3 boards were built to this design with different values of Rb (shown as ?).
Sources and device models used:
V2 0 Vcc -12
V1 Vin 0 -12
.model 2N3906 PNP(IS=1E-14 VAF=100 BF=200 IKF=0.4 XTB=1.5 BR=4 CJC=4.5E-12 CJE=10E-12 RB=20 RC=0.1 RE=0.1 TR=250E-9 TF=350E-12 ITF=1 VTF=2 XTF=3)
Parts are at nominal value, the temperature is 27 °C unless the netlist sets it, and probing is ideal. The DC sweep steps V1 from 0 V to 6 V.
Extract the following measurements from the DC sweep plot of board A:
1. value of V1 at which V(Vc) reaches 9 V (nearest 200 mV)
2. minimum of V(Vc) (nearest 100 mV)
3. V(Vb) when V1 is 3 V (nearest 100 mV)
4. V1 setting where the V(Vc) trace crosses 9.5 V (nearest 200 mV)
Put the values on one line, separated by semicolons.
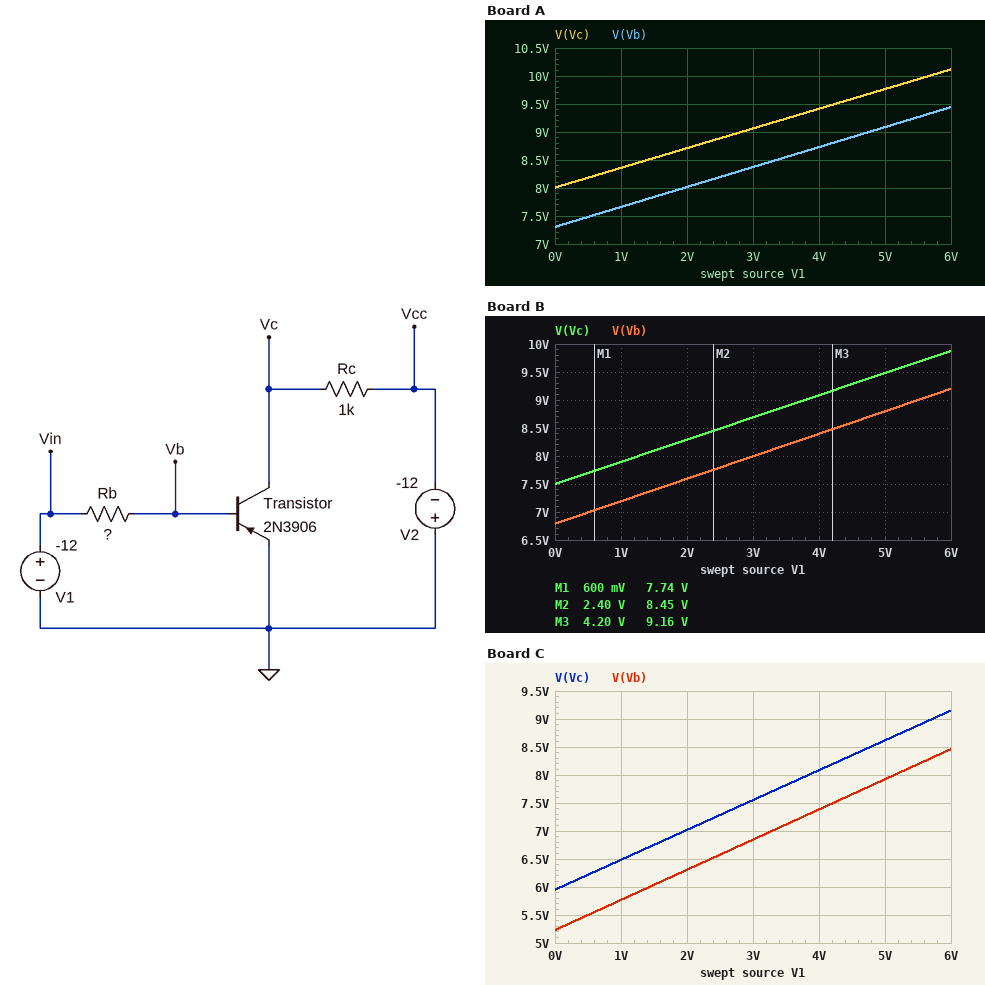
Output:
2.8 V; 8.0 V; 8.4 V; 4.2 V
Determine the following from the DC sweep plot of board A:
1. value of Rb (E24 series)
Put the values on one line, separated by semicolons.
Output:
9.1 kΩ
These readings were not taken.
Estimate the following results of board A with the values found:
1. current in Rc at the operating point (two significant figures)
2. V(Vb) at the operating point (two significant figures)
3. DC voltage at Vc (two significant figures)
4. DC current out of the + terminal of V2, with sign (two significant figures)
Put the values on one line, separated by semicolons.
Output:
8.2 mA; 3.0 V; 3.8 V; -8.2 mA
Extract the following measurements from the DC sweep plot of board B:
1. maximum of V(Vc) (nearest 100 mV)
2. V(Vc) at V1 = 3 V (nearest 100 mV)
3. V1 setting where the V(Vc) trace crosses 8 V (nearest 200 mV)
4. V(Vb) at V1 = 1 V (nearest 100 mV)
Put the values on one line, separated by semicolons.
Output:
9.9 V; 8.7 V; 1.2 V; 7.2 V
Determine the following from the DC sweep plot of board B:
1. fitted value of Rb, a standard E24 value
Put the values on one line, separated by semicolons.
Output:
7.5 kΩ
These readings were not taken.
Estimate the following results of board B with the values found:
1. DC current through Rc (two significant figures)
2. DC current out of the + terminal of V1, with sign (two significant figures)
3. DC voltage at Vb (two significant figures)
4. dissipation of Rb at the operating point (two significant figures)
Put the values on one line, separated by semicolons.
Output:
9.3 mA; -1.9 mA; 2.0 V; 26 mW
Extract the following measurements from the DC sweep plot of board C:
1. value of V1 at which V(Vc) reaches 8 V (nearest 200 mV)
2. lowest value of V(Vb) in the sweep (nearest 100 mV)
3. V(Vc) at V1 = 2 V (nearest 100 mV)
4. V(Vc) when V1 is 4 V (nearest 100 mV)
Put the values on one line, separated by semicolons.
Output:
3.8 V; 5.2 V; 7.0 V; 8.1 V
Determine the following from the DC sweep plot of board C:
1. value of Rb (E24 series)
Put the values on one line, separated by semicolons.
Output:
4.3 kΩ
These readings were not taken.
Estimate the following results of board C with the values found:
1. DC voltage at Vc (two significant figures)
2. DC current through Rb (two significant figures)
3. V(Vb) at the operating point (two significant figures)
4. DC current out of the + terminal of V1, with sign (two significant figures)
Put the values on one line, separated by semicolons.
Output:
61 mV; 2.6 mA; -710 mV; -2.6 mA
